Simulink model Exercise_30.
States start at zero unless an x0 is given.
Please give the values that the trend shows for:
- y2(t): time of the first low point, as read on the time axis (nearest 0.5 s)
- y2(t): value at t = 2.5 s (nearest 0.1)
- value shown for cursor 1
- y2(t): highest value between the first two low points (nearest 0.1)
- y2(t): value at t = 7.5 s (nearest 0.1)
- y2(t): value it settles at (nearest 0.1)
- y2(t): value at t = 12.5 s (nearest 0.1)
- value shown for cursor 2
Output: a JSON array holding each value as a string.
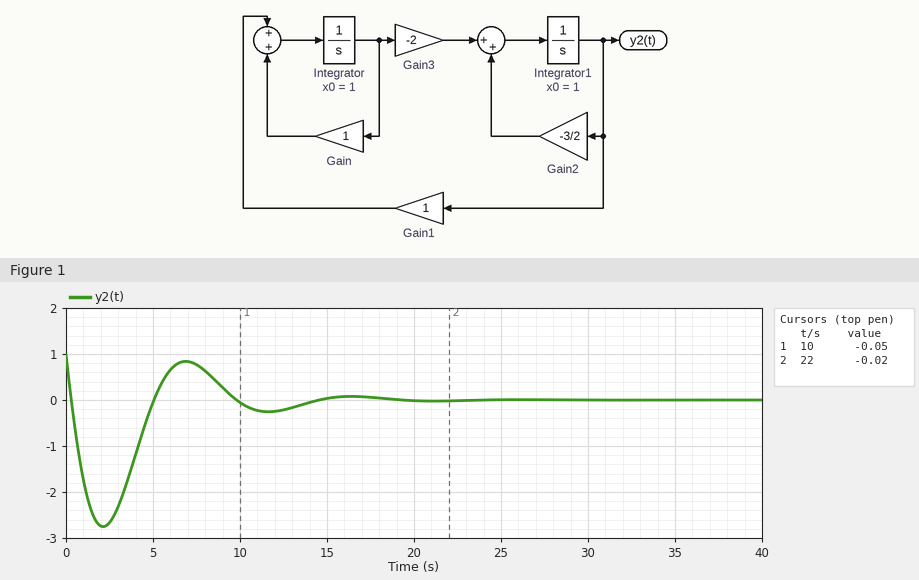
["2.0 s", "-2.7", "-0.05", "0.8", "0.8", "0.0", "-0.2", "-0.02"]
